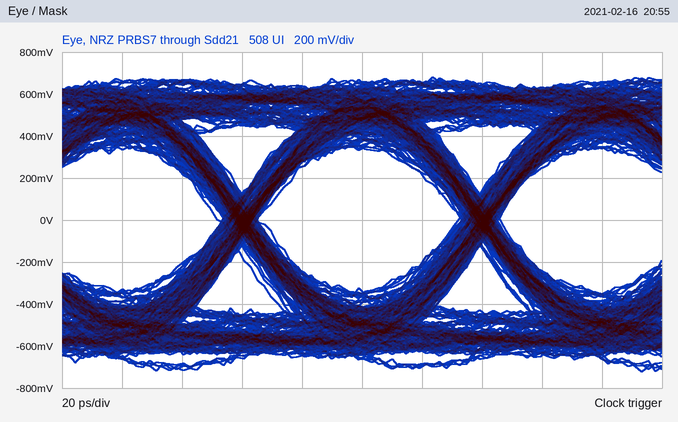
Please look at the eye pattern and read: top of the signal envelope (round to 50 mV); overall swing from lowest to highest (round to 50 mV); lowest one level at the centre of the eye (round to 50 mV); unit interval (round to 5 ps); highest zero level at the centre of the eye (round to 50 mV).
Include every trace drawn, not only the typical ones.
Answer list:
700 mV
1.40 V
350 mV
80 ps
-350 mV
